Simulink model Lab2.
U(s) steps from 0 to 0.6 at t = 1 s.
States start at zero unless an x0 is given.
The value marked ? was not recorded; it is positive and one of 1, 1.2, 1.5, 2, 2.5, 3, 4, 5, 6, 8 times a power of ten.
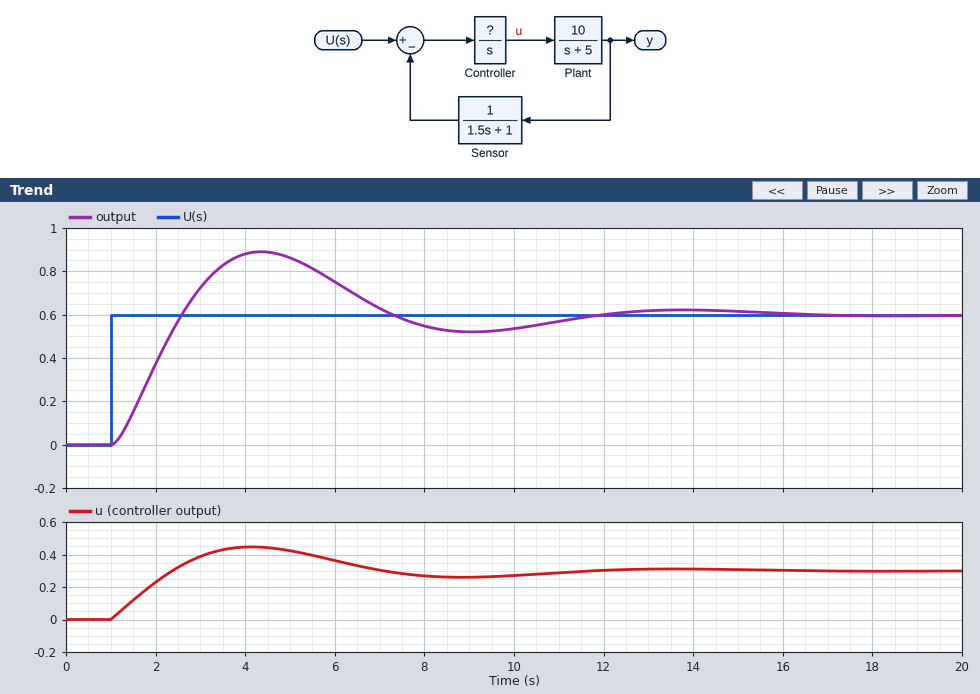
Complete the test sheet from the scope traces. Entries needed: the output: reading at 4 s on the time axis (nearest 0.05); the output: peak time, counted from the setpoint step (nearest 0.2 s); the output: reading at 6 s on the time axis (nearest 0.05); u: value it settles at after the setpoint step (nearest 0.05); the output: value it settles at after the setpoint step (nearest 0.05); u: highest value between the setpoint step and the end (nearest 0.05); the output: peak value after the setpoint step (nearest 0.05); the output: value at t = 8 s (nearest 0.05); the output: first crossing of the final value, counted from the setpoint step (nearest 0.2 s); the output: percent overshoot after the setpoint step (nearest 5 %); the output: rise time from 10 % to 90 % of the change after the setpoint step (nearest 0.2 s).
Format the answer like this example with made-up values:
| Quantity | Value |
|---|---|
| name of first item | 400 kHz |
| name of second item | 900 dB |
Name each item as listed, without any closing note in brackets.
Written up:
| Quantity | Value |
|---|---|
| the output: reading at 4 s on the time axis | 0.90 |
| the output: peak time, counted from the setpoint step | 3.4 s |
| the output: reading at 6 s on the time axis | 0.75 |
| u: value it settles at after the setpoint step | 0.30 |
| the output: value it settles at after the setpoint step | 0.60 |
| u: highest value between the setpoint step and the end | 0.45 |
| the output: peak value after the setpoint step | 0.90 |
| the output: value at t = 8 s | 0.55 |
| the output: first crossing of the final value, counted from the setpoint step | 1.6 s |
| the output: percent overshoot after the setpoint step | 50 % |
| the output: rise time from 10 % to 90 % of the change after the setpoint step | 1.2 s |
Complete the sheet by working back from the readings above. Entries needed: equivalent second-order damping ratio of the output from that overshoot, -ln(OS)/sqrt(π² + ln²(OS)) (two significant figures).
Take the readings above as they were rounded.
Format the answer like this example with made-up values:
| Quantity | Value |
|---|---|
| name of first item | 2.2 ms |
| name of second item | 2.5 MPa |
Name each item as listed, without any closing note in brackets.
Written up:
| Quantity | Value |
|---|---|
| equivalent second-order damping ratio of the output from that overshoot, -ln(OS)/sqrt(π² + ln²(OS)) | 0.22 |
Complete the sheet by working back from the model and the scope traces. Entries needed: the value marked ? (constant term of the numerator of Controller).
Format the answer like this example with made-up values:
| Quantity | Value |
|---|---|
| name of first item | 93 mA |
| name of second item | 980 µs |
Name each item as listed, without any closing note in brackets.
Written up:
| Quantity | Value |
|---|---|
| the value marked ? | 0.4 |
